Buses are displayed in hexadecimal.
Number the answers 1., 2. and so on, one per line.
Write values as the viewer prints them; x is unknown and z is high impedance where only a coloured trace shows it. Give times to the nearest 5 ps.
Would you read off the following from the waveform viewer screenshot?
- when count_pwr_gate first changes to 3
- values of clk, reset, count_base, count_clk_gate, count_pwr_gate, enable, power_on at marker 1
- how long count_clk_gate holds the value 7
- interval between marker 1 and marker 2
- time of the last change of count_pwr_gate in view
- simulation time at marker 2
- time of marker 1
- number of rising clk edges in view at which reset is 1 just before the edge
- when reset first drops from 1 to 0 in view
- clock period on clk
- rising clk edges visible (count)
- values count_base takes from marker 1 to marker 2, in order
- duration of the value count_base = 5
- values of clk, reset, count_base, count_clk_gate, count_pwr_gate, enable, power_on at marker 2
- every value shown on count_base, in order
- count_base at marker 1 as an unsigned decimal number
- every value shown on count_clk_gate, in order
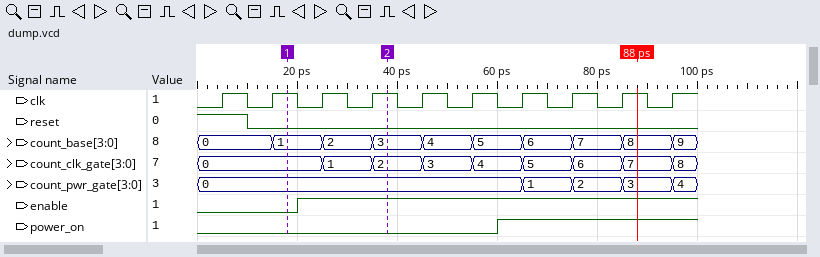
1. 85 ps
2. clk=1, reset=0, count_base=1, count_clk_gate=0, count_pwr_gate=0, enable=0, power_on=0
3. 10 ps
4. 20 ps
5. 95 ps
6. 40 ps
7. 20 ps
8. 1
9. 10 ps
10. 10 ps
11. 10
12. 1, 2, 3
13. 10 ps
14. clk=1, reset=0, count_base=3, count_clk_gate=2, count_pwr_gate=0, enable=1, power_on=0
15. 0, 1, 2, 3, 4, 5, 6, 7, 8, 9
16. 1
17. 0, 1, 2, 3, 4, 5, 6, 7, 8
